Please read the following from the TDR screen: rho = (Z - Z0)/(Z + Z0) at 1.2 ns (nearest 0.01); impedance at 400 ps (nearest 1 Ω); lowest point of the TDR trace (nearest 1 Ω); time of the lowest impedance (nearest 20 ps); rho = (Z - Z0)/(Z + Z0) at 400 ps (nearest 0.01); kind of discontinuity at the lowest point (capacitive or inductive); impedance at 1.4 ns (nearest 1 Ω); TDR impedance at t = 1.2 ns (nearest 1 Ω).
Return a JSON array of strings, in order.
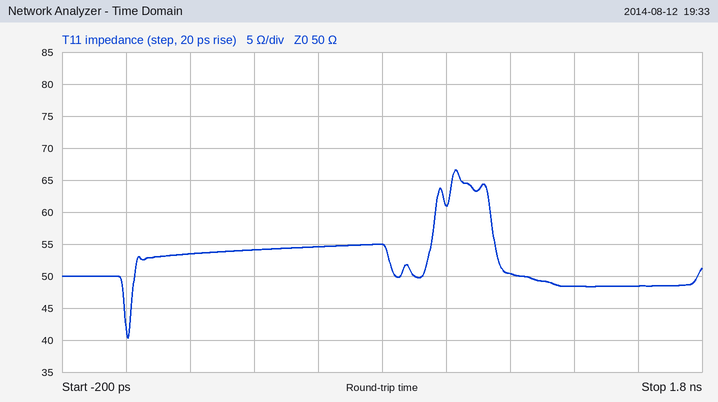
["0.00", "54 Ω", "40 Ω", "0 ps", "+0.04", "capacitive", "48 Ω", "50 Ω"]
